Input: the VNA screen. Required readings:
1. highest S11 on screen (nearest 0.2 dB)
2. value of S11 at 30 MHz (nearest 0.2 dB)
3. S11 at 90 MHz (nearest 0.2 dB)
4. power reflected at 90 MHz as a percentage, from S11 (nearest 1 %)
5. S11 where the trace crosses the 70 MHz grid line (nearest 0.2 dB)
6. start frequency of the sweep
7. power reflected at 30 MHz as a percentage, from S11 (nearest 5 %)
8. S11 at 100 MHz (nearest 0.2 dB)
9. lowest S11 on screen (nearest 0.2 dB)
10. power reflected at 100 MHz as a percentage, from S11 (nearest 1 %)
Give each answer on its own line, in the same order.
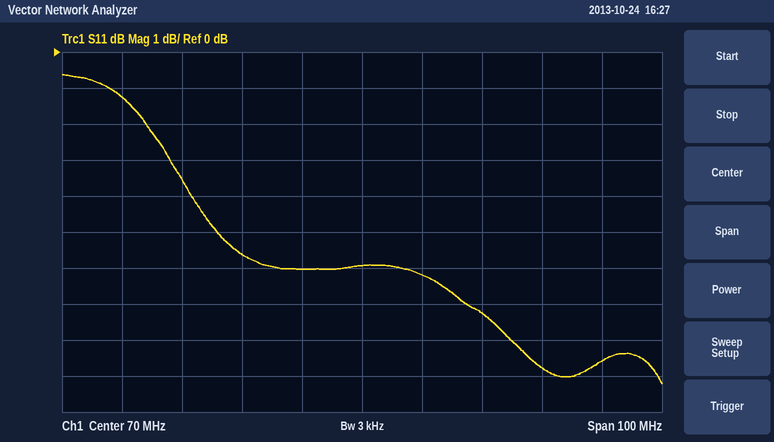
-0.6 dB
-1.2 dB
-7.2 dB
19 %
-6.0 dB
20 MHz
75 %
-8.8 dB
-9.2 dB
13 %
